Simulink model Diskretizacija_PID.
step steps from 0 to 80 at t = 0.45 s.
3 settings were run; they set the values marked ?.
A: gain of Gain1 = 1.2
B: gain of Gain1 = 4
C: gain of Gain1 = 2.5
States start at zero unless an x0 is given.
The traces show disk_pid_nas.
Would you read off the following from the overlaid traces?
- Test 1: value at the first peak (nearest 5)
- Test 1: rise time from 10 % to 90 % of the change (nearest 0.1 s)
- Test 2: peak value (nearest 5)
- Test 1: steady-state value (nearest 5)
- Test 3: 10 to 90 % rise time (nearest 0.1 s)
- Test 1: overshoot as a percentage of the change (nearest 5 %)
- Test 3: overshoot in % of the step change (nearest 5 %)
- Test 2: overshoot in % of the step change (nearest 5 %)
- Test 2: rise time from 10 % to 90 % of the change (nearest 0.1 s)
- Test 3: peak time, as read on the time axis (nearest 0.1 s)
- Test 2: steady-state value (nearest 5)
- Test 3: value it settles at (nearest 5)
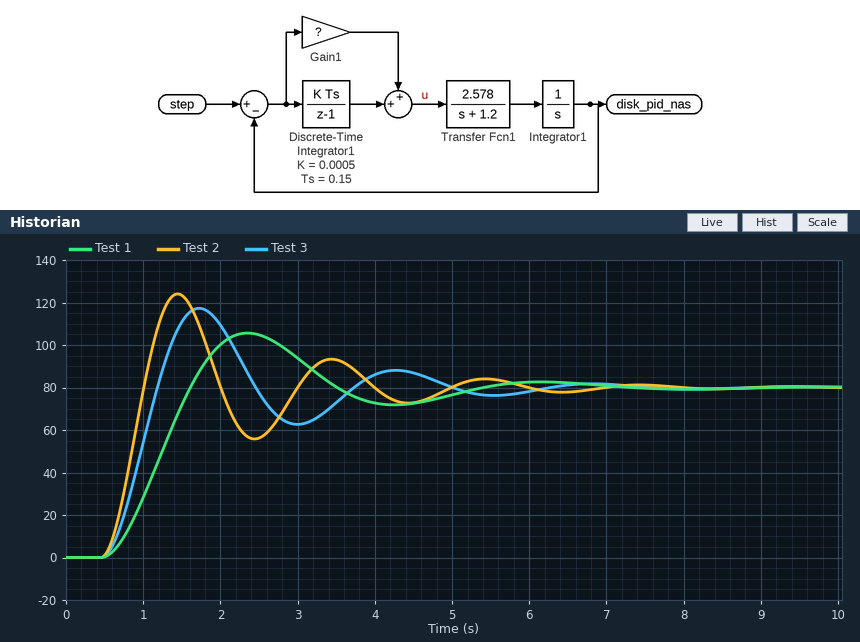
105
0.8 s
125
80
0.5 s
30 %
45 %
55 %
0.4 s
1.7 s
80
80
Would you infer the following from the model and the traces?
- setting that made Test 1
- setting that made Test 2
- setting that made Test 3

A
B
C
